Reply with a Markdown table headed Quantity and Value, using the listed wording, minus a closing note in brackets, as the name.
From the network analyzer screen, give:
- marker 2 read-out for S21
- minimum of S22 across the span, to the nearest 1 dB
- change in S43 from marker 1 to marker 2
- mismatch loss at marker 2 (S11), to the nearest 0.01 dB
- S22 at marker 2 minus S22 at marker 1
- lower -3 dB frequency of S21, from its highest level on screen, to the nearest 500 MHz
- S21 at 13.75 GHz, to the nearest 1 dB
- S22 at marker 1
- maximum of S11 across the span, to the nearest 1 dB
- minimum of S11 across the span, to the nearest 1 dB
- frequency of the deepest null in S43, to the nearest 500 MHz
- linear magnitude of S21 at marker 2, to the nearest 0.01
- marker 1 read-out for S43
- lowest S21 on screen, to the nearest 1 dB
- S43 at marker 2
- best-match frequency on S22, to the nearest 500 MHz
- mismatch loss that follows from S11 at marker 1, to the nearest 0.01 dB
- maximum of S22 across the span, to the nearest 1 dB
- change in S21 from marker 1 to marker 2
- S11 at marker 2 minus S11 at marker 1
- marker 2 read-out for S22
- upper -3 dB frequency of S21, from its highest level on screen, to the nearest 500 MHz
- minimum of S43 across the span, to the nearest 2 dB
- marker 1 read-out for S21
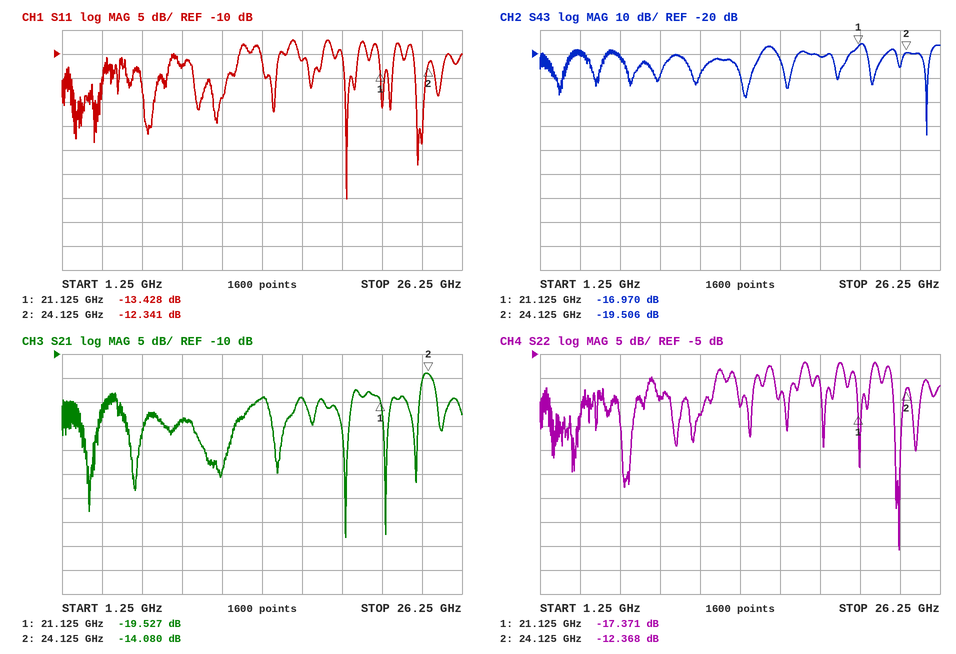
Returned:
| Quantity | Value |
|---|---|
| marker 2 read-out for S21 | -14.080 dB |
| minimum of S22 across the span, to the nearest 1 dB | -46 dB |
| change in S43 from marker 1 to marker 2 | -2.536 dB |
| mismatch loss at marker 2 (S11), to the nearest 0.01 dB | 0.26 dB |
| S22 at marker 2 minus S22 at marker 1 | 5.003 dB |
| lower -3 dB frequency of S21, from its highest level on screen, to the nearest 500 MHz | 23.5 GHz |
| S21 at 13.75 GHz, to the nearest 1 dB | -19 dB |
| S22 at marker 1 | -17.371 dB |
| maximum of S11 across the span, to the nearest 1 dB | -7 dB |
| minimum of S11 across the span, to the nearest 1 dB | -40 dB |
| frequency of the deepest null in S43, to the nearest 500 MHz | 25.5 GHz |
| linear magnitude of S21 at marker 2, to the nearest 0.01 | 0.20 |
| marker 1 read-out for S43 | -16.970 dB |
| lowest S21 on screen, to the nearest 1 dB | -48 dB |
| S43 at marker 2 | -19.506 dB |
| best-match frequency on S22, to the nearest 500 MHz | 23.5 GHz |
| mismatch loss that follows from S11 at marker 1, to the nearest 0.01 dB | 0.20 dB |
| maximum of S22 across the span, to the nearest 1 dB | -7 dB |
| change in S21 from marker 1 to marker 2 | 5.447 dB |
| S11 at marker 2 minus S11 at marker 1 | 1.087 dB |
| marker 2 read-out for S22 | -12.368 dB |
| upper -3 dB frequency of S21, from its highest level on screen, to the nearest 500 MHz | 24.5 GHz |
| minimum of S43 across the span, to the nearest 2 dB | -54 dB |
| marker 1 read-out for S21 | -19.527 dB |
